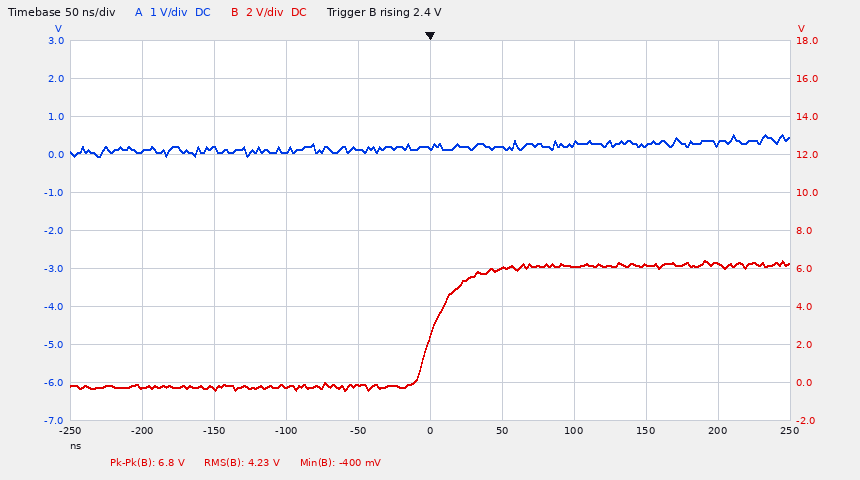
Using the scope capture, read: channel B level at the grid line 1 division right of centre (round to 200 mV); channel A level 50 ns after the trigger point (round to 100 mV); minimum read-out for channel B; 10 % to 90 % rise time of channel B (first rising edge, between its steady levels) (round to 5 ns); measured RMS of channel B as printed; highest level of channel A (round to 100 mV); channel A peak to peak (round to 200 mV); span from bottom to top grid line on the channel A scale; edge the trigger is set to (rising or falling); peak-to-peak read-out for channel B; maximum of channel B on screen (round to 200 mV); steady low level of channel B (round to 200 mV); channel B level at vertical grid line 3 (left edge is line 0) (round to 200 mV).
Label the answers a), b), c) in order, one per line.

a) 6.0 V
b) 200 mV
c) -400 mV
d) 35 ns
e) 4.23 V
f) 500 mV
g) 600 mV
h) 10 V
i) rising
j) 6.8 V
k) 6.4 V
l) -200 mV
m) -200 mV
